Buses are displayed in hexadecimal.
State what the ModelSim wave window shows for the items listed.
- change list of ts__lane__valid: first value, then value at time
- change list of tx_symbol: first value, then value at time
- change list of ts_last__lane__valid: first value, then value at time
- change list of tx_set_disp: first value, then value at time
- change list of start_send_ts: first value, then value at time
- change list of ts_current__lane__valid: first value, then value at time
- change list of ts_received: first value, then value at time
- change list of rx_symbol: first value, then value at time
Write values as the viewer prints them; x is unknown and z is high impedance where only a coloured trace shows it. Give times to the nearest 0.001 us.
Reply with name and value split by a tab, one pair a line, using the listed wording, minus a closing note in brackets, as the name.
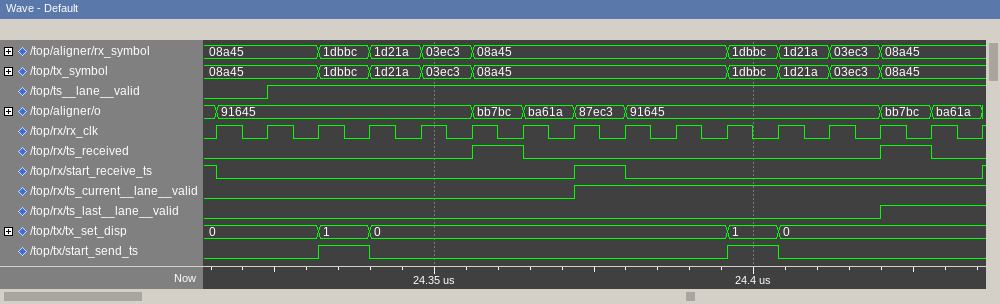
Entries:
change list of ts__lane__valid: first value, then value at time	0, 1 at 24.324 us
change list of tx_symbol: first value, then value at time	08a45, 1dbbc at 24.332 us, 1d21a at 24.34 us, 03ec3 at 24.348 us, 08a45 at 24.356 us, 1dbbc at 24.396 us, 1d21a at 24.404 us, 03ec3 at 24.412 us, 08a45 at 24.42 us
change list of ts_last__lane__valid: first value, then value at time	0, 1 at 24.42 us
change list of tx_set_disp: first value, then value at time	0, 1 at 24.332 us, 0 at 24.34 us, 1 at 24.396 us, 0 at 24.404 us
change list of start_send_ts: first value, then value at time	0, 1 at 24.332 us, 0 at 24.34 us, 1 at 24.396 us, 0 at 24.404 us
change list of ts_current__lane__valid: first value, then value at time	0, 1 at 24.372 us
change list of ts_received: first value, then value at time	0, 1 at 24.356 us, 0 at 24.364 us, 1 at 24.42 us, 0 at 24.428 us
change list of rx_symbol: first value, then value at time	08a45, 1dbbc at 24.332 us, 1d21a at 24.34 us, 03ec3 at 24.348 us, 08a45 at 24.356 us, 1dbbc at 24.396 us, 1d21a at 24.404 us, 03ec3 at 24.412 us, 08a45 at 24.42 us
